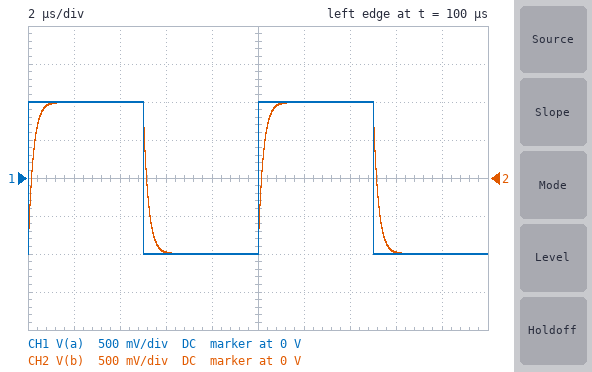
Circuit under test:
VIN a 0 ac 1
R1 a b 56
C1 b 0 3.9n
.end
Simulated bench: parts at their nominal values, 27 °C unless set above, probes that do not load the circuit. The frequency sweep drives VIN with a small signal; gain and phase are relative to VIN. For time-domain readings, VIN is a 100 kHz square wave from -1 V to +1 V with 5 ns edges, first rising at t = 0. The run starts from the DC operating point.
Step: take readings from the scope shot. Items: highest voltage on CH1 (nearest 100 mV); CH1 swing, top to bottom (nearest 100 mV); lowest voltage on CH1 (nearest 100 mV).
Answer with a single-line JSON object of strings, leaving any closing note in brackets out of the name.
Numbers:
{"highest voltage on CH1": "1.0 V", "CH1 swing, top to bottom": "2.0 V", "lowest voltage on CH1": "-1.0 V"}
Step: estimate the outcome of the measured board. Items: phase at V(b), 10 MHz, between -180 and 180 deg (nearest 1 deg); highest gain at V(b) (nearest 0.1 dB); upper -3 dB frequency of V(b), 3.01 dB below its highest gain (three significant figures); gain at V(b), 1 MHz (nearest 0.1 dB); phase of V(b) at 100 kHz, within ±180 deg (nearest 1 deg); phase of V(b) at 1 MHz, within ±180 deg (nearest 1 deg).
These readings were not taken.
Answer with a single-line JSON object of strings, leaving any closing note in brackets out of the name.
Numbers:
{"phase at V(b), 10 MHz, between -180 and 180 deg": "-86 deg", "highest gain at V(b)": "0 dB", "upper -3 dB frequency of V(b), 3.01 dB below its highest gain": "729 kHz", "gain at V(b), 1 MHz": "-4.6 dB", "phase of V(b) at 100 kHz, within ±180 deg": "-8 deg", "phase of V(b) at 1 MHz, within ±180 deg": "-54 deg"}
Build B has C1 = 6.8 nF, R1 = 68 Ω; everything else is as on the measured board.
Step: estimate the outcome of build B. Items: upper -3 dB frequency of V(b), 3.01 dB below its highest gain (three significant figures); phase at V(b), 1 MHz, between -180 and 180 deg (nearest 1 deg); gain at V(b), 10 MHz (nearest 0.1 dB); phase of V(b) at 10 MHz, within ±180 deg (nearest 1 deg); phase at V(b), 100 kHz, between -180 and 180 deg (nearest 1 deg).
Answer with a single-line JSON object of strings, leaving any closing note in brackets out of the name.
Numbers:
{"upper -3 dB frequency of V(b), 3.01 dB below its highest gain": "344 kHz", "phase at V(b), 1 MHz, between -180 and 180 deg": "-71 deg", "gain at V(b), 10 MHz": "-29.3 dB", "phase of V(b) at 10 MHz, within ±180 deg": "-88 deg", "phase at V(b), 100 kHz, between -180 and 180 deg": "-16 deg"}
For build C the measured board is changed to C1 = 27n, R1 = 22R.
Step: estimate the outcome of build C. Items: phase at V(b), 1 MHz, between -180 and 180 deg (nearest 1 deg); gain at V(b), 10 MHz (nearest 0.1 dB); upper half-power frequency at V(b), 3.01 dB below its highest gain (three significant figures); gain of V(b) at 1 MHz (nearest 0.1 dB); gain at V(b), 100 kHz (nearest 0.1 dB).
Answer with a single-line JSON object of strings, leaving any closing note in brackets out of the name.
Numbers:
{"phase at V(b), 1 MHz, between -180 and 180 deg": "-75 deg", "gain at V(b), 10 MHz": "-31.4 dB", "upper half-power frequency at V(b), 3.01 dB below its highest gain": "268 kHz", "gain of V(b) at 1 MHz": "-11.7 dB", "gain at V(b), 100 kHz": "-0.6 dB"}
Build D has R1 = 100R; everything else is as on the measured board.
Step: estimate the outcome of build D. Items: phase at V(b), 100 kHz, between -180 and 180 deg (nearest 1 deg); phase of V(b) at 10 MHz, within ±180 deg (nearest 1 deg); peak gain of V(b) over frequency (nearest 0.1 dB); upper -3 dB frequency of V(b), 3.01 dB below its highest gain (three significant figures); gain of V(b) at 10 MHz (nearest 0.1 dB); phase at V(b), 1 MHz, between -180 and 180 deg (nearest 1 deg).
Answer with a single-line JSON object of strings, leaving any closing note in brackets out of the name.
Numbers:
{"phase at V(b), 100 kHz, between -180 and 180 deg": "-14 deg", "phase of V(b) at 10 MHz, within ±180 deg": "-88 deg", "peak gain of V(b) over frequency": "0 dB", "upper -3 dB frequency of V(b), 3.01 dB below its highest gain": "408 kHz", "gain of V(b) at 10 MHz": "-27.8 dB", "phase at V(b), 1 MHz, between -180 and 180 deg": "-68 deg"}
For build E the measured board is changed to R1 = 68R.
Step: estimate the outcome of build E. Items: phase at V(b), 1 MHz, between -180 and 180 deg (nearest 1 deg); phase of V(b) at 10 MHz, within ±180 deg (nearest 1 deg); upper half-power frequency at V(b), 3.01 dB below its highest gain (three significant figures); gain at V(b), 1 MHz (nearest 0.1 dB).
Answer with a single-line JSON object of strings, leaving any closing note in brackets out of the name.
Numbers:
{"phase at V(b), 1 MHz, between -180 and 180 deg": "-59 deg", "phase of V(b) at 10 MHz, within ±180 deg": "-87 deg", "upper half-power frequency at V(b), 3.01 dB below its highest gain": "600 kHz", "gain at V(b), 1 MHz": "-5.8 dB"}
